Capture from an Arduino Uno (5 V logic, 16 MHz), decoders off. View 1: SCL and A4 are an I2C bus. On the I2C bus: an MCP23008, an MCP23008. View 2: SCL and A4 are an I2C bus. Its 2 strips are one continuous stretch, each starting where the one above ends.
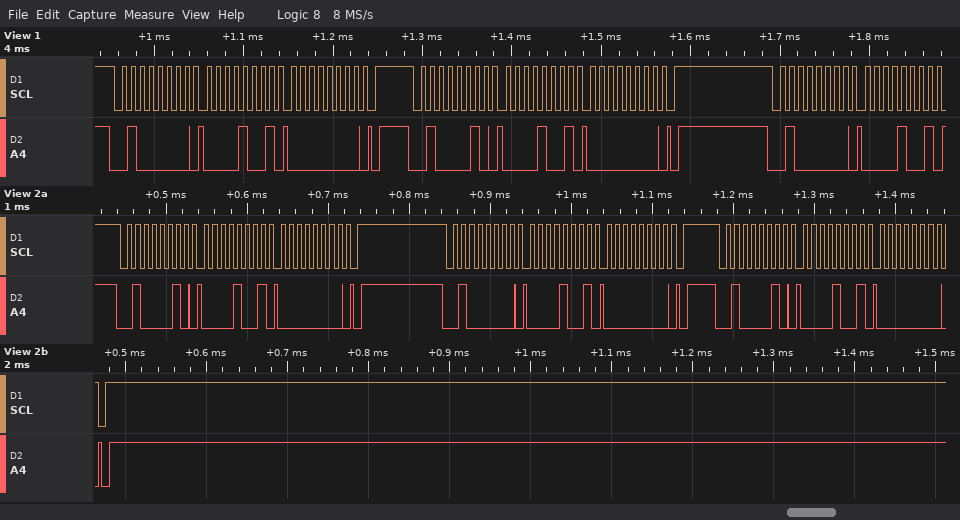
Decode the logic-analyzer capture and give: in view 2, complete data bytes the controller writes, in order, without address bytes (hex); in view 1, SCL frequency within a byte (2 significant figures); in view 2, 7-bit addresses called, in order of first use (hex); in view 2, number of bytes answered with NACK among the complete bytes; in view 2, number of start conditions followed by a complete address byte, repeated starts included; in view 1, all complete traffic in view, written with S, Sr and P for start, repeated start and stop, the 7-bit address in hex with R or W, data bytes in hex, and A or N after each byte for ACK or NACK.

09 00 09 00 09 00
100 kHz
0x21 0x20
0
3
S 20W A 09 A 00 A P S 21W A 09 A 00 A P S 20W A 09 A
